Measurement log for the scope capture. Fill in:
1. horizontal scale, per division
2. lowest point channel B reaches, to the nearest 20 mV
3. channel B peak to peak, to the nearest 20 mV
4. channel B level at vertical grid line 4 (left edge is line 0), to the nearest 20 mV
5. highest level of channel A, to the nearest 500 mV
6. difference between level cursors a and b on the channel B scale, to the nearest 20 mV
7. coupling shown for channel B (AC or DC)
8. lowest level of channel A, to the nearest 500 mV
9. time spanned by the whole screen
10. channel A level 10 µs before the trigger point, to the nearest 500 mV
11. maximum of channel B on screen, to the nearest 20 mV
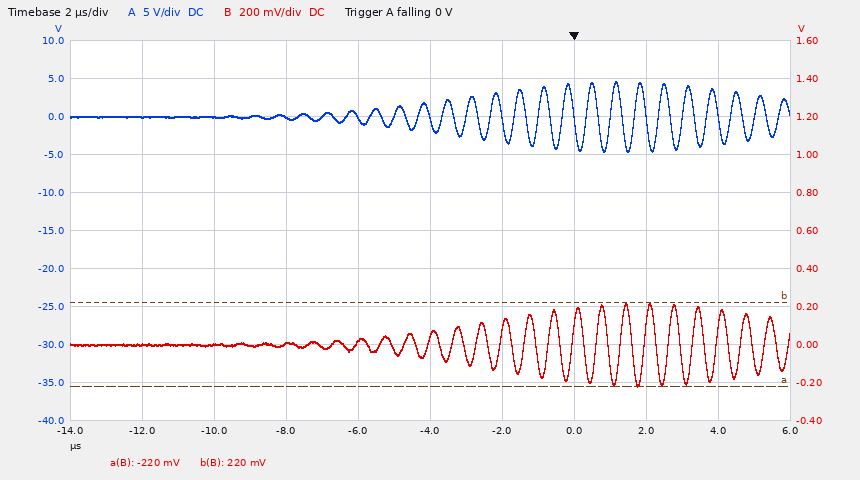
2 µs
-220 mV
440 mV
20 mV
4.5 V
440 mV
DC
-4.5 V
20 µs
0.0 V
220 mV
